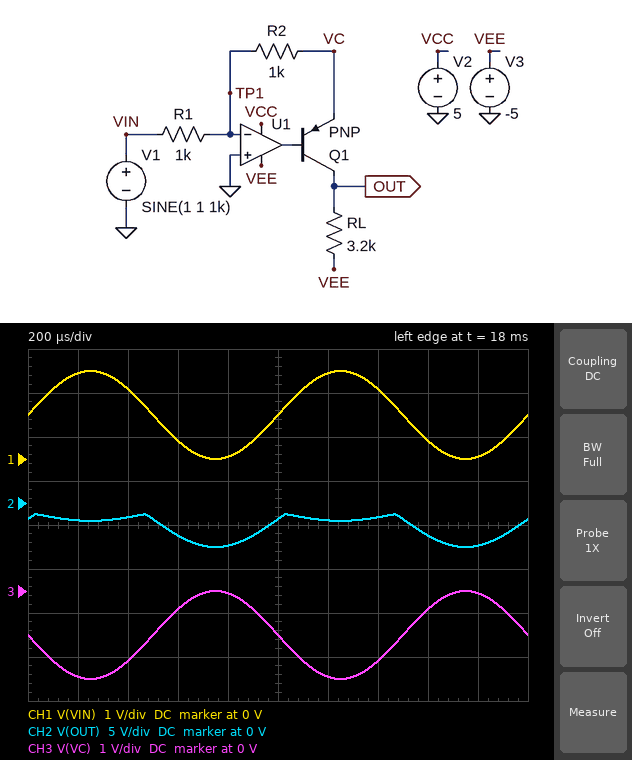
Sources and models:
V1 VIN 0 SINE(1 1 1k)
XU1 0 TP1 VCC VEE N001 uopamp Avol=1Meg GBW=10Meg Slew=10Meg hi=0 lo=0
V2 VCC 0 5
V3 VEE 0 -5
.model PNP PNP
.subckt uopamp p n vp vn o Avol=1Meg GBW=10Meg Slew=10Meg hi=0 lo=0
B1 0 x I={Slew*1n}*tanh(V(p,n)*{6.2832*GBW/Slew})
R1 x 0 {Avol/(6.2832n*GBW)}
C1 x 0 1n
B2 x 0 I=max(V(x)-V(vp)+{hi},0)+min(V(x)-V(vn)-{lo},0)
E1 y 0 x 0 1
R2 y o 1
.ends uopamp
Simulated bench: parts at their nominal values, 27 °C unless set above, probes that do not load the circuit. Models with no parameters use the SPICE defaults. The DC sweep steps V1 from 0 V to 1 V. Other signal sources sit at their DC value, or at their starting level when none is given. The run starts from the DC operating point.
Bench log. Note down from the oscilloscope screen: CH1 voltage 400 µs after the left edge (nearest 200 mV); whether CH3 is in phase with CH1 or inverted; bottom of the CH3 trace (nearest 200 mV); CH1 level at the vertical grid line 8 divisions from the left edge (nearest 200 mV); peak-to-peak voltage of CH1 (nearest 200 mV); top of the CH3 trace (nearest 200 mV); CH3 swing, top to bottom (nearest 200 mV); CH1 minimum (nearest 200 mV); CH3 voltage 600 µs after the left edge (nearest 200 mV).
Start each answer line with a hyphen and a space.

- 1.6 V
- inverted
- -2.0 V
- 400 mV
- 2.0 V
- 0 V
- 2.0 V
- 0 V
- -400 mV
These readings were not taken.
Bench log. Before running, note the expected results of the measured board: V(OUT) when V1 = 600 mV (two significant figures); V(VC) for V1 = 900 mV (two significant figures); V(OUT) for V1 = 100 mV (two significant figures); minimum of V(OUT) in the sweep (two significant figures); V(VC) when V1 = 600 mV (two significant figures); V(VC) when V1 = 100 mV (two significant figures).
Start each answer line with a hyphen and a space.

- -3.1 V
- -900 mV
- -4.7 V
- -5.0 V
- -600 mV
- -100 mV
